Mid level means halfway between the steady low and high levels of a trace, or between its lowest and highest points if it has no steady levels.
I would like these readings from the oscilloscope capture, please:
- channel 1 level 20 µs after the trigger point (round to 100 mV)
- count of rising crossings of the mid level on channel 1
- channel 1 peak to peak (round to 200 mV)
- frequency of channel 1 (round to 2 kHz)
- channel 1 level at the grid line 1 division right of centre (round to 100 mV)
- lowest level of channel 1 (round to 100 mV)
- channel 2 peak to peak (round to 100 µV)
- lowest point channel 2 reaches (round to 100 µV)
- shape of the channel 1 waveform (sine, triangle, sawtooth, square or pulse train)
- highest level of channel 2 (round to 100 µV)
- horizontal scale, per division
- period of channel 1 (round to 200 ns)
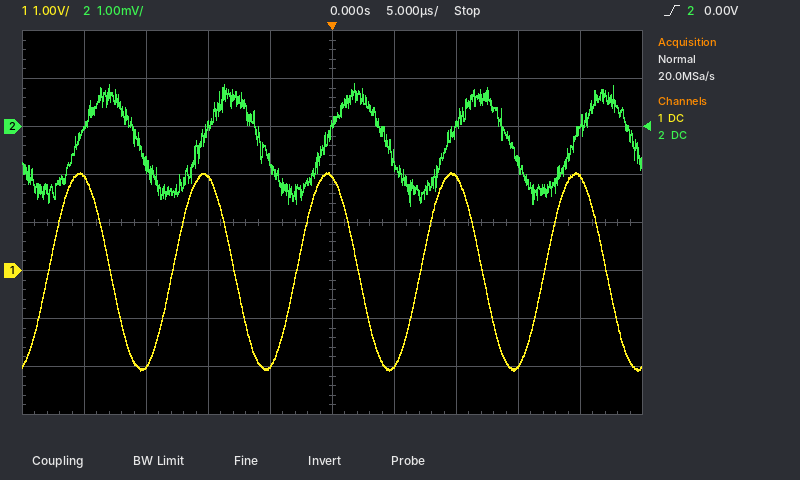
1.9 V
5
4.2 V
100 kHz
-2.0 V
-2.1 V
2.5 mV
-1.6 mV
sine
900 µV
5 µs
10.0 µs
